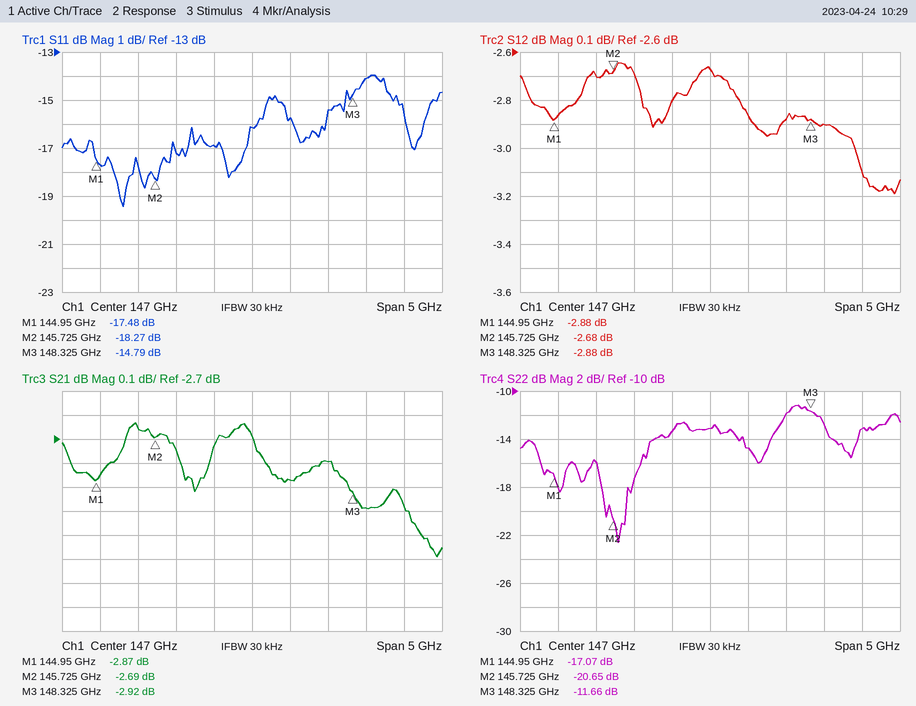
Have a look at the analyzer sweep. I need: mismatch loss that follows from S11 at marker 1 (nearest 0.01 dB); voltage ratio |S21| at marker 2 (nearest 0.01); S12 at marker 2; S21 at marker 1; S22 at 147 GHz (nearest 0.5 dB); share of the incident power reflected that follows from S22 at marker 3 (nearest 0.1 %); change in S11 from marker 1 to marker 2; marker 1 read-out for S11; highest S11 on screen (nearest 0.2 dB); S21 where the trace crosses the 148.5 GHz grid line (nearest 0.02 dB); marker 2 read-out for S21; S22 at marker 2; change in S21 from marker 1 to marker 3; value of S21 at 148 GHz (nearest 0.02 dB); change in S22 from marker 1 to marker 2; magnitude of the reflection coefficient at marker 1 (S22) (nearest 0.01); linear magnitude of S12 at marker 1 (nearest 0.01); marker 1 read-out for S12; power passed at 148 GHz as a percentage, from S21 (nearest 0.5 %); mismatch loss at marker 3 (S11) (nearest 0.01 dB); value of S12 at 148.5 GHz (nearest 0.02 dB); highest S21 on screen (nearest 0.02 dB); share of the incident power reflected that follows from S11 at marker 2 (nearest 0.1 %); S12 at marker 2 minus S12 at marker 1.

0.08 dB
0.73
-2.68 dB
-2.87 dB
-13.0 dB
6.8 %
-0.79 dB
-17.48 dB
-14.0 dB
-2.98 dB
-2.69 dB
-20.65 dB
-0.05 dB
-2.80 dB
-3.58 dB
0.14
0.72
-2.88 dB
52.5 %
0.15 dB
-2.90 dB
-2.64 dB
1.5 %
0.20 dB
